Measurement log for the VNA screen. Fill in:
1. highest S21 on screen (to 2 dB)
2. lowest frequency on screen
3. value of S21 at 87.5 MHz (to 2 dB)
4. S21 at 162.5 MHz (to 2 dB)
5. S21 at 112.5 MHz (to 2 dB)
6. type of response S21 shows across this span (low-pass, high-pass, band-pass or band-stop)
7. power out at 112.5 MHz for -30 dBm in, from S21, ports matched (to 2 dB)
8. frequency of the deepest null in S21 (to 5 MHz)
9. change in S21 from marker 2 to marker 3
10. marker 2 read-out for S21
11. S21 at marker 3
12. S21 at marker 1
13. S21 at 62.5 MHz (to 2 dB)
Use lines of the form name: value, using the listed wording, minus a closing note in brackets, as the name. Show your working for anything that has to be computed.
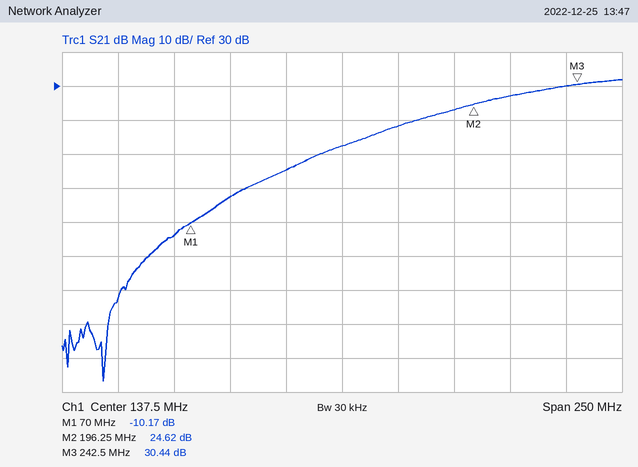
highest S21 on screen: 32 dB
lowest frequency on screen: 12.5 MHz
value of S21 at 87.5 MHz: -2 dB
S21 at 162.5 MHz: 18 dB
S21 at 112.5 MHz: 6 dB
type of response S21 shows across this span: high-pass
power out at 112.5 MHz for -30 dBm in, from S21, ports matched: -30 dBm + (6 dB) = -24 dBm
frequency of the deepest null in S21: 30 MHz
change in S21 from marker 2 to marker 3: 30.44 − (24.62) = 5.82 dB
marker 2 read-out for S21: 24.62 dB
S21 at marker 3: 30.44 dB
S21 at marker 1: -10.17 dB
S21 at 62.5 MHz: -14 dB
